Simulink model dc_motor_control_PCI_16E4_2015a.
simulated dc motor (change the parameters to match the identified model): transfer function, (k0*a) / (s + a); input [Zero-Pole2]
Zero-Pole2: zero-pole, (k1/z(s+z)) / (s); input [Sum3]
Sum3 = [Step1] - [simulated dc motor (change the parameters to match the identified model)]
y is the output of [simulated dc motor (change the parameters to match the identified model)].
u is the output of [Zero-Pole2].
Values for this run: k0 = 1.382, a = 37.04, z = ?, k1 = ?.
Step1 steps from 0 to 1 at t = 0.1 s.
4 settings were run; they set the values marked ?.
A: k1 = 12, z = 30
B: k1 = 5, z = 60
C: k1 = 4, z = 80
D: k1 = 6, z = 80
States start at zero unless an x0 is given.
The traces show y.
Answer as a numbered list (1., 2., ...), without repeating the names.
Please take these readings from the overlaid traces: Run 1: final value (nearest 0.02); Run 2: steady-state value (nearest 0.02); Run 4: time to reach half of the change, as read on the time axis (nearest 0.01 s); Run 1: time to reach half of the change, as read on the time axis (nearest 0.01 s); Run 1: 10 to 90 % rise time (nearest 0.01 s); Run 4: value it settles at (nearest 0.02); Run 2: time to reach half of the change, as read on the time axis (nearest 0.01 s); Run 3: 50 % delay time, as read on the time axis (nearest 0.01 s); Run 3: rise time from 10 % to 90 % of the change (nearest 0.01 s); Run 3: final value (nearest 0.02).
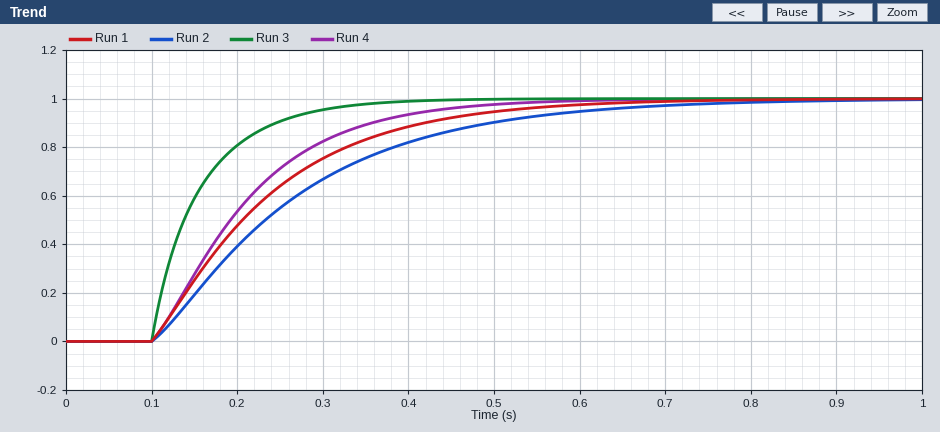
1. 1.00
2. 1.00
3. 0.19 s
4. 0.21 s
5. 0.30 s
6. 1.00
7. 0.23 s
8. 0.14 s
9. 0.14 s
10. 1.00
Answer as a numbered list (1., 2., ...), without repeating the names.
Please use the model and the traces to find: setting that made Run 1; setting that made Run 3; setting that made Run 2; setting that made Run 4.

1. B
2. A
3. C
4. D
